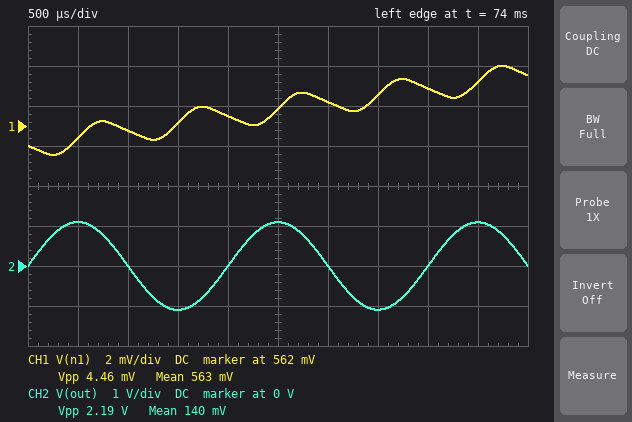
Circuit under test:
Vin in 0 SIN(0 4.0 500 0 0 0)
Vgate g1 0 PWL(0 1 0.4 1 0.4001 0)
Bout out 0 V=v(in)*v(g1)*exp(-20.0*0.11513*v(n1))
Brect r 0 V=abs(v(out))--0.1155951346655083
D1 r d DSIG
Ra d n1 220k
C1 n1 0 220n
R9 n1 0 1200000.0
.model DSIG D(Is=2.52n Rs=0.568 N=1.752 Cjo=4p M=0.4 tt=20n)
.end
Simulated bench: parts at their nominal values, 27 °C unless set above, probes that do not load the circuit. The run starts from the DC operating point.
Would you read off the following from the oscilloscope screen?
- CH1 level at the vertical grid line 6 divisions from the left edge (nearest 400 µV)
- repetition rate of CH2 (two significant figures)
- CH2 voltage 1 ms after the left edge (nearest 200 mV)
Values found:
563.2 mV
500 Hz
0 V
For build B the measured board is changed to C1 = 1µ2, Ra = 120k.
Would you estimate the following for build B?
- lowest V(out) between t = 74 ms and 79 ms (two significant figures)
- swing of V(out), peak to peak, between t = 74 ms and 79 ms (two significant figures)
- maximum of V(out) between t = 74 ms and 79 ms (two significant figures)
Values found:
-1.4 V
2.9 V
1.4 V
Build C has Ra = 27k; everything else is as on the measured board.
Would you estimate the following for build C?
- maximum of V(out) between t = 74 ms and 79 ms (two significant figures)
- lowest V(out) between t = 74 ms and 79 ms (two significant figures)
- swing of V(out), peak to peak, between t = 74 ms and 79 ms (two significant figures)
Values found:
900 mV
-900 mV
1.8 V
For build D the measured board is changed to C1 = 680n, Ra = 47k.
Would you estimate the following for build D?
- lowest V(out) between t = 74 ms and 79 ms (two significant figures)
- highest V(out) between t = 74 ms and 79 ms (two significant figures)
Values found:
-980 mV
980 mV
